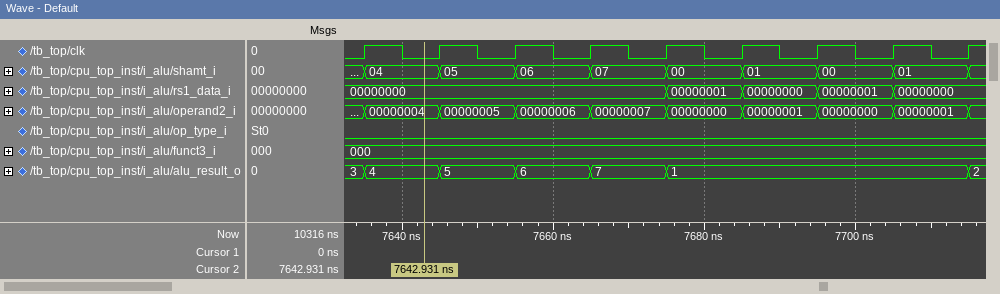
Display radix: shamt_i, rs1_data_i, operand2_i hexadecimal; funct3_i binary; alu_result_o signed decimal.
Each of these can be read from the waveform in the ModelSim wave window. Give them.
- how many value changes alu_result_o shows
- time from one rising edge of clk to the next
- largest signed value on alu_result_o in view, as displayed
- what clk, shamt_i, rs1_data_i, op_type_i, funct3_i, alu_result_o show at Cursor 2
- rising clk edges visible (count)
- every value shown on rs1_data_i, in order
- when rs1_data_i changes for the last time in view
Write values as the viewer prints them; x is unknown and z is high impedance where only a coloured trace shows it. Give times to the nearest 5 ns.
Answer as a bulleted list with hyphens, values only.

- 6
- 10 ns
- 7
- clk=0, shamt_i=04, rs1_data_i=00000000, op_type_i=0, funct3_i=000, alu_result_o=4
- 9
- 00000000, 00000001, 00000000, 00000001, 00000000
- 7705 ns
